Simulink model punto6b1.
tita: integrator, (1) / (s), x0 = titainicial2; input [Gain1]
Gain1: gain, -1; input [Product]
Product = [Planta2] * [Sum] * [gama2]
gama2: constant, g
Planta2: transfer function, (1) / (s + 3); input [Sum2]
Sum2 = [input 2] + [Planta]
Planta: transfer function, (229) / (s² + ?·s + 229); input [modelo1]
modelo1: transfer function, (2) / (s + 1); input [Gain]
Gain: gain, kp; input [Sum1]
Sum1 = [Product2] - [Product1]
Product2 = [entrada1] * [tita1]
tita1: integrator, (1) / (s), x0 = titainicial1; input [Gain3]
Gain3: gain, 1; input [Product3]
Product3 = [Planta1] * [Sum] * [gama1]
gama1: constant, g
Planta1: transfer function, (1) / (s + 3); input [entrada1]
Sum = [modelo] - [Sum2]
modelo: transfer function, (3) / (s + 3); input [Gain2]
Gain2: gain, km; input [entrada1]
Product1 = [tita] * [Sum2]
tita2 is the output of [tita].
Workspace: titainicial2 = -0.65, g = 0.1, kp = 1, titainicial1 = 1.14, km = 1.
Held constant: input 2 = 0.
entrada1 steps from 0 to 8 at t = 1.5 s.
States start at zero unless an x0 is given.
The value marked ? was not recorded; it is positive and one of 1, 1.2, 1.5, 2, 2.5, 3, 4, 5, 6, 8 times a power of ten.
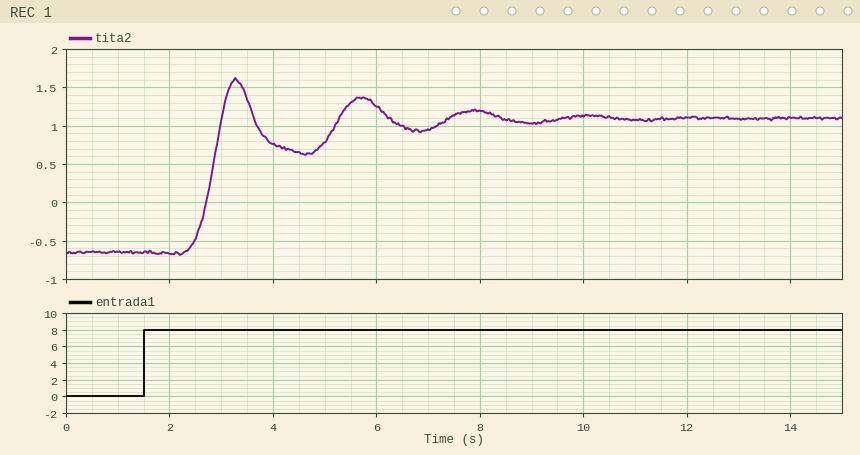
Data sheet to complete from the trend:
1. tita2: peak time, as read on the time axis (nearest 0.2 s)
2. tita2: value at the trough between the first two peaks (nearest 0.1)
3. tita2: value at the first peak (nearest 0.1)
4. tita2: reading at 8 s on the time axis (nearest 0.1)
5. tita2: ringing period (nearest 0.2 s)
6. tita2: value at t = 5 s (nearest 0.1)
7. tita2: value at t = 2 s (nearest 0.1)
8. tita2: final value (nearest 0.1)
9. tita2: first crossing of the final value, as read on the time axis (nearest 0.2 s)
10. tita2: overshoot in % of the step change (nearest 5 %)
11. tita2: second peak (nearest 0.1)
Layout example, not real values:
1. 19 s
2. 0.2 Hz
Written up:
1. 3.2 s
2. 0.6
3. 1.6
4. 1.2
5. 2.4 s
6. 0.8
7. -0.7
8. 1.1
9. 3.0 s
10. 30 %
11. 1.4
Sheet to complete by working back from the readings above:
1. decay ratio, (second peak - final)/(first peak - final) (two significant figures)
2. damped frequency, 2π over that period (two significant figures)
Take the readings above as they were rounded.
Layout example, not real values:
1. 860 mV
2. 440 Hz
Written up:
1. 0.60
2. 2.6 rad/s
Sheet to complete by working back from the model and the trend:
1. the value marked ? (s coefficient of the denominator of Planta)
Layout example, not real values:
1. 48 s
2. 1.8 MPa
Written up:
1. 60
